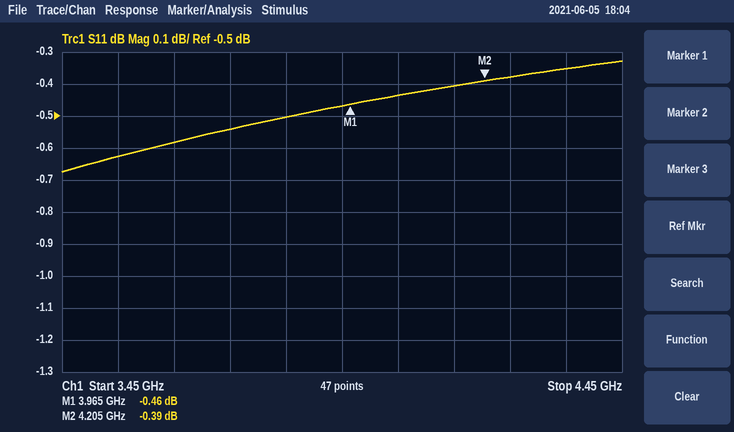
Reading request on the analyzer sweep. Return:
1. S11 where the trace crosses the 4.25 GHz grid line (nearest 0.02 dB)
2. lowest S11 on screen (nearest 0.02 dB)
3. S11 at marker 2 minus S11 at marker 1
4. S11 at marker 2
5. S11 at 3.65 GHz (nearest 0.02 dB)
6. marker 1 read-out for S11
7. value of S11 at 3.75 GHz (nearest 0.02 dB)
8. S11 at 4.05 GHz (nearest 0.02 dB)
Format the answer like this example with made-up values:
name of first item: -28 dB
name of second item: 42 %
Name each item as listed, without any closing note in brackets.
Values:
S11 where the trace crosses the 4.25 GHz grid line: -0.38 dB
lowest S11 on screen: -0.68 dB
S11 at marker 2 minus S11 at marker 1: 0.07 dB
S11 at marker 2: -0.39 dB
S11 at 3.65 GHz: -0.58 dB
marker 1 read-out for S11: -0.46 dB
value of S11 at 3.75 GHz: -0.54 dB
S11 at 4.05 GHz: -0.44 dB
